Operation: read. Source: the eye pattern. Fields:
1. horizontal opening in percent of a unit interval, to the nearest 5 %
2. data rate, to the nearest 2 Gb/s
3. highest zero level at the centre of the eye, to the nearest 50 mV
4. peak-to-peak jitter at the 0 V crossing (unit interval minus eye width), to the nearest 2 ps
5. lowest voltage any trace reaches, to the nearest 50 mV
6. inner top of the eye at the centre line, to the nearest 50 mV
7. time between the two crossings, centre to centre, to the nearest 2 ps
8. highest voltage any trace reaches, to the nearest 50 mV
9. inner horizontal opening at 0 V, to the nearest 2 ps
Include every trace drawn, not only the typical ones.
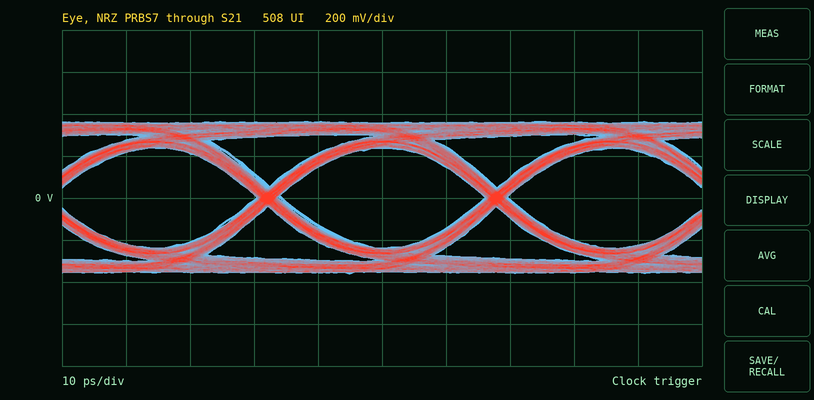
90 %
28 Gb/s
-250 mV
4 ps
-350 mV
250 mV
36 ps
350 mV
32 ps
